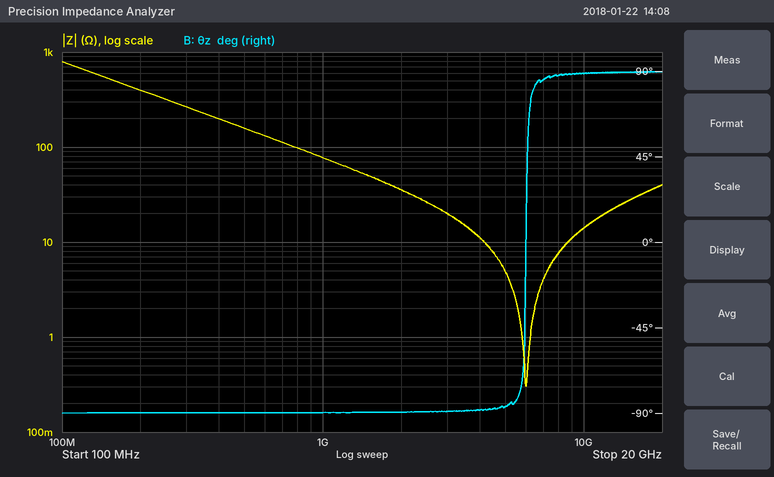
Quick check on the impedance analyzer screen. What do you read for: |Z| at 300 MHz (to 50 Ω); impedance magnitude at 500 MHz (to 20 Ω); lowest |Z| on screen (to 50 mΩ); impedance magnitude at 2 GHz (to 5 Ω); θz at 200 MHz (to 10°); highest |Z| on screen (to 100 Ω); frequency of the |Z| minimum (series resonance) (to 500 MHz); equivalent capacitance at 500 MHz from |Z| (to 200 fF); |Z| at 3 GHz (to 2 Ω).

250 Ω
160 Ω
300 mΩ
35 Ω
-90°
800 Ω
6.0 GHz
2.0 pF
20 Ω
